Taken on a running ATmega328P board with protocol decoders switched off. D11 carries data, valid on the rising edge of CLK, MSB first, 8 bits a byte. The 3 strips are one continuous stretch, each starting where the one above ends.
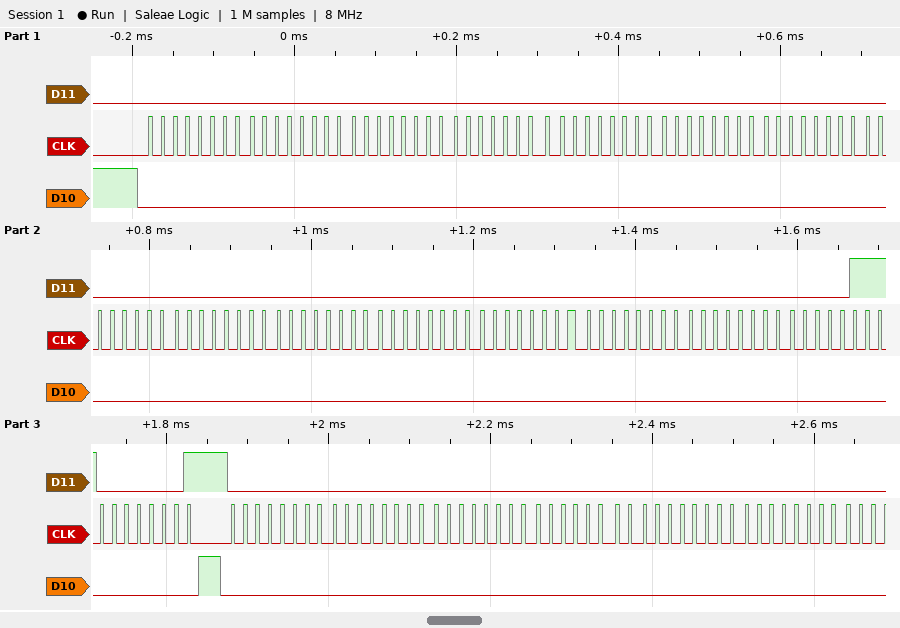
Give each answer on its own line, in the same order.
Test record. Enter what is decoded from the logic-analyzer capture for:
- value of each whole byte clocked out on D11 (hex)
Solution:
00 00 00 00 00 00 00 00 00 00 00 00 00 00 07 01 00 00 00 00 00 00
